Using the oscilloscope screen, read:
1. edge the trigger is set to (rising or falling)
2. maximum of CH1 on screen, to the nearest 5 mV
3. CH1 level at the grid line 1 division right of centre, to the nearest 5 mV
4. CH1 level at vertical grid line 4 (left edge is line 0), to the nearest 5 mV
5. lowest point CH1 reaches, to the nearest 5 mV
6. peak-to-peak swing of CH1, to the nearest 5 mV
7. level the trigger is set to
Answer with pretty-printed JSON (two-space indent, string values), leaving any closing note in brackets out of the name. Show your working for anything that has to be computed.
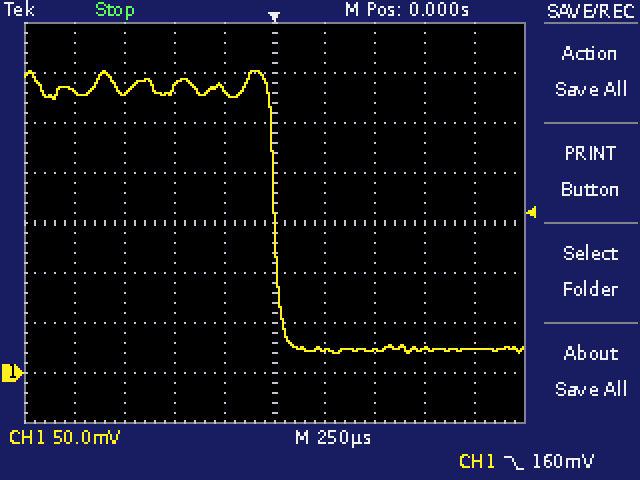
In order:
{
  "edge the trigger is set to": "falling",
  "maximum of CH1 on screen, to the nearest 5 mV": "300 mV",
  "CH1 level at the grid line 1 division right of centre, to the nearest 5 mV": "25 mV",
  "CH1 level at vertical grid line 4 (left edge is line 0), to the nearest 5 mV": "285 mV",
  "lowest point CH1 reaches, to the nearest 5 mV": "20 mV",
  "peak-to-peak swing of CH1, to the nearest 5 mV": "300 mV − (20 mV) = 280 mV",
  "level the trigger is set to": "160 mV"
}
